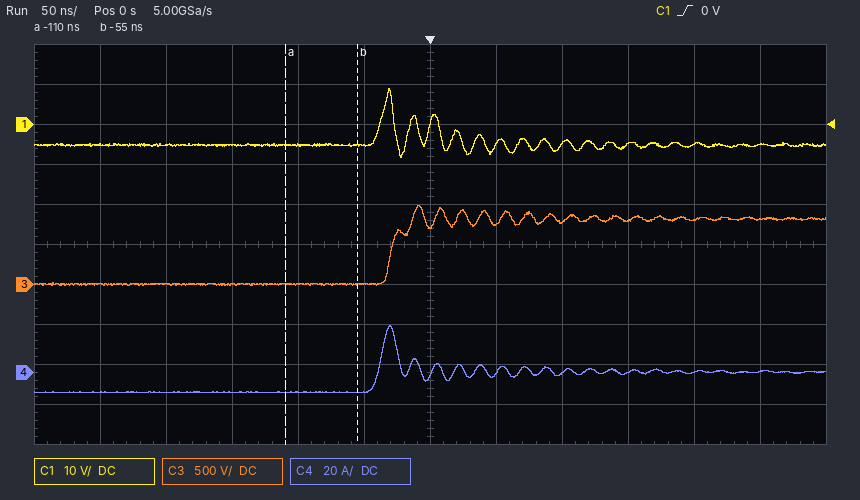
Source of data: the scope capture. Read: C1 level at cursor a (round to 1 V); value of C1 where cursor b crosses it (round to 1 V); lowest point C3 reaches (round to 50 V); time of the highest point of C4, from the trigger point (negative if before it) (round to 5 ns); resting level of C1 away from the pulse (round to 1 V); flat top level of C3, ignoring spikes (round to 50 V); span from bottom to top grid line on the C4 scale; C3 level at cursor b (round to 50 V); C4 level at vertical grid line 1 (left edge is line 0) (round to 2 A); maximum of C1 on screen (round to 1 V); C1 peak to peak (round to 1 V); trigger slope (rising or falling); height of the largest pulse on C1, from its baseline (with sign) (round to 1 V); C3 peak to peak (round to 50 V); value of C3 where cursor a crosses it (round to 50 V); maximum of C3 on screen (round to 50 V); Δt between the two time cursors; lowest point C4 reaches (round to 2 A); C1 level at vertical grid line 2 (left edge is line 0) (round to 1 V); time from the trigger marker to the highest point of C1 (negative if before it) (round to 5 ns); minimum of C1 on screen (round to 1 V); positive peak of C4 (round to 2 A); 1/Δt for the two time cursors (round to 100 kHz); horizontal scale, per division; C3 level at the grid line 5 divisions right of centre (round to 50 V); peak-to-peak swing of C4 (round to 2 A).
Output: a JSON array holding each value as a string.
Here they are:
["-5 V", "-5 V", "0 V", "-30 ns", "-5 V", "800 V", "200 A", "0 V", "-10 A", "9 V", "17 V", "rising", "+14 V", "1.00 kV", "0 V", "1.00 kV", "55 ns", "-10 A", "-5 V", "-30 ns", "-8 V", "24 A", "18.2 MHz", "50 ns", "800 V", "34 A"]
